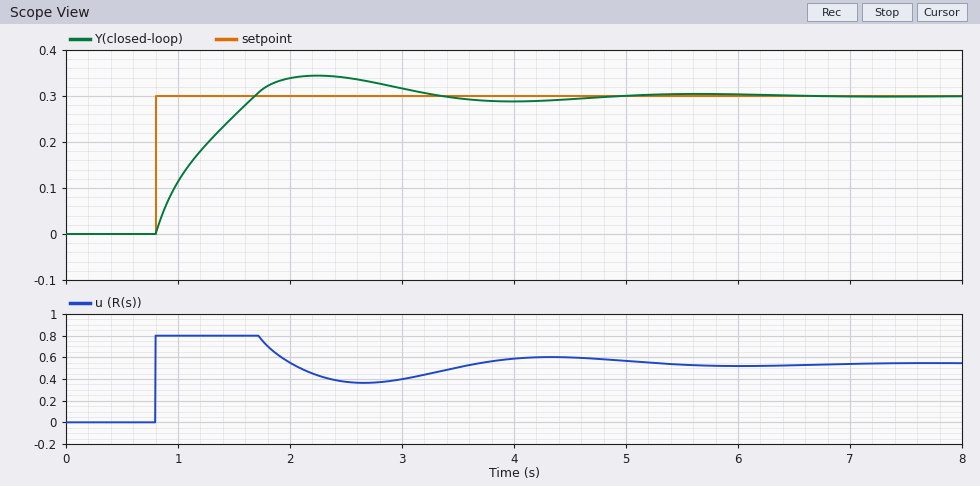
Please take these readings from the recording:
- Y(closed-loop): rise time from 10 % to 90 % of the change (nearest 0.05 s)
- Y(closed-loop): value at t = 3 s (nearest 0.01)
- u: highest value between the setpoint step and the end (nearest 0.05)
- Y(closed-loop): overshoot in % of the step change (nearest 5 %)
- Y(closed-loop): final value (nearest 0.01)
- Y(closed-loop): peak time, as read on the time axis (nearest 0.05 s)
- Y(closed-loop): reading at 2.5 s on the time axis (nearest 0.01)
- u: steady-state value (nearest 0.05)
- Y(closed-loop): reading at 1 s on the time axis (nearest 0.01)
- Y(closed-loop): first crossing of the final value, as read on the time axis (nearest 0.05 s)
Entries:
0.70 s
0.32
0.80
15 %
0.30
2.25 s
0.34
0.55
0.11
1.70 s
